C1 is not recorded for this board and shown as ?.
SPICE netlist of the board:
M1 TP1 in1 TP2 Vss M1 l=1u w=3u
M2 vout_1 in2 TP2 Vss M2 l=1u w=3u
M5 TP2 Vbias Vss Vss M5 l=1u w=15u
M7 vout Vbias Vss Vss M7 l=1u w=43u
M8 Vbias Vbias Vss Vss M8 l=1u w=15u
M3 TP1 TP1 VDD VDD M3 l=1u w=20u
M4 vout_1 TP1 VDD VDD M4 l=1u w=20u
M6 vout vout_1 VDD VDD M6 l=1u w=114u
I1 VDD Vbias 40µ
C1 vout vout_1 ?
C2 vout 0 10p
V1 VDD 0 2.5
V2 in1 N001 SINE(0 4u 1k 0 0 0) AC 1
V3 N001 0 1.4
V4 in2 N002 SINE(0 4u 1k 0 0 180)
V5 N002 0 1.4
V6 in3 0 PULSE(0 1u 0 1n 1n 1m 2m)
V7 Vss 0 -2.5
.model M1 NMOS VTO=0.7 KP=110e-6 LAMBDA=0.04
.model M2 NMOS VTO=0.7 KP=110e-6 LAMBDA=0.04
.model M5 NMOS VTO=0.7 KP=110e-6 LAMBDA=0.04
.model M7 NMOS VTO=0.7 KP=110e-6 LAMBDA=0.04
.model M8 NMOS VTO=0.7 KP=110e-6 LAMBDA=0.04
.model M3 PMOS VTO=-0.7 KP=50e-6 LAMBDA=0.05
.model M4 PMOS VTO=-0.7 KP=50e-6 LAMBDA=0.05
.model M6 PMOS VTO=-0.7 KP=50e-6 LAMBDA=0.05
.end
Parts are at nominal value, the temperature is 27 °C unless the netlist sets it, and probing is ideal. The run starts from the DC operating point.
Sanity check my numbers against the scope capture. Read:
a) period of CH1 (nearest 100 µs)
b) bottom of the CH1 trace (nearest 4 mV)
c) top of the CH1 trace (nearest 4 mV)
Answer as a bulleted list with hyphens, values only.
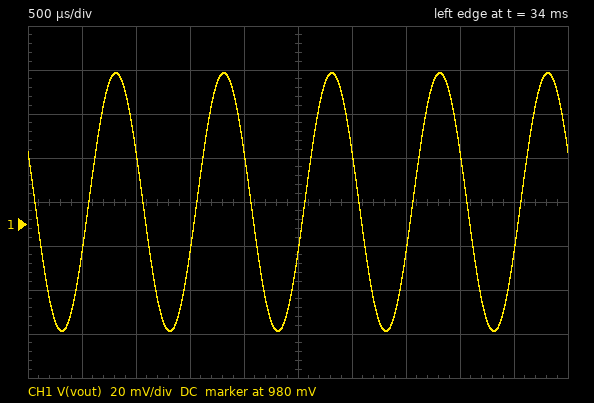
- 1.0 ms
- 932 mV
- 1.048 V
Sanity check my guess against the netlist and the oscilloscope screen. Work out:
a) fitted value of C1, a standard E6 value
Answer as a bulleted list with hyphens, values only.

- 1 pF
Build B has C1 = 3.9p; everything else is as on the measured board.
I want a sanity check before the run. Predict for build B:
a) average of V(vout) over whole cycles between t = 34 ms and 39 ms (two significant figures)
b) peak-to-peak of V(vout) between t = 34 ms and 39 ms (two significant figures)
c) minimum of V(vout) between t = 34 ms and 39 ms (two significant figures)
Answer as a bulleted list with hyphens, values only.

- 990 mV
- 67 mV
- 960 mV
